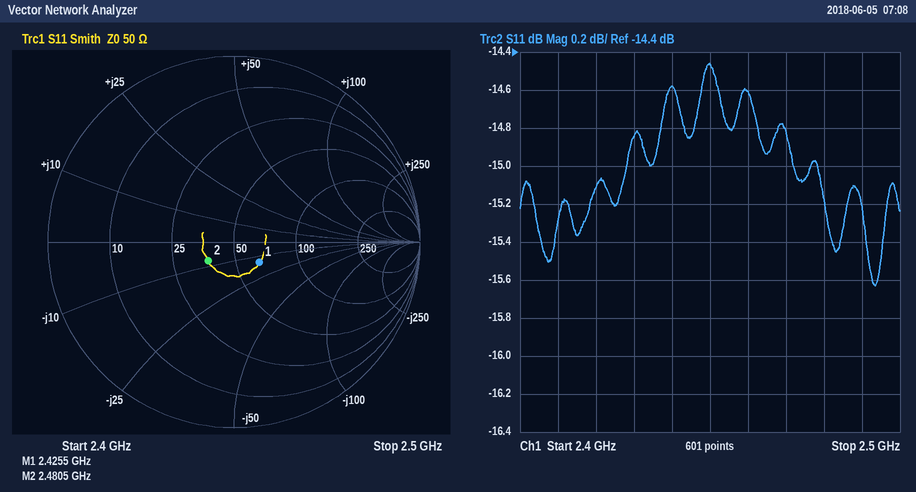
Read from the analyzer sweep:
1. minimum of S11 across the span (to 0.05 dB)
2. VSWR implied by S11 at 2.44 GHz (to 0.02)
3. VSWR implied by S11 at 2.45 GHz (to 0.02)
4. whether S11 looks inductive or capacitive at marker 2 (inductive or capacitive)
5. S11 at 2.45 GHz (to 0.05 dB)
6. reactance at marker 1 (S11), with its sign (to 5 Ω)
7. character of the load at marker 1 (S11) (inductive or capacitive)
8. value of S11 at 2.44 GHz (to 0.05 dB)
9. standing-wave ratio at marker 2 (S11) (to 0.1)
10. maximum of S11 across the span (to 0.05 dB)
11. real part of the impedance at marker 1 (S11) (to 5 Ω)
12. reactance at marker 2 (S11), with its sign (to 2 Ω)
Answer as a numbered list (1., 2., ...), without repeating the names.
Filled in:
1. -15.65 dB
2. 1.46
3. 1.46
4. capacitive
5. -14.45 dB
6. -15 Ω
7. capacitive
8. -14.60 dB
9. 1.4
10. -14.45 dB
11. 65 Ω
12. -8 Ω
